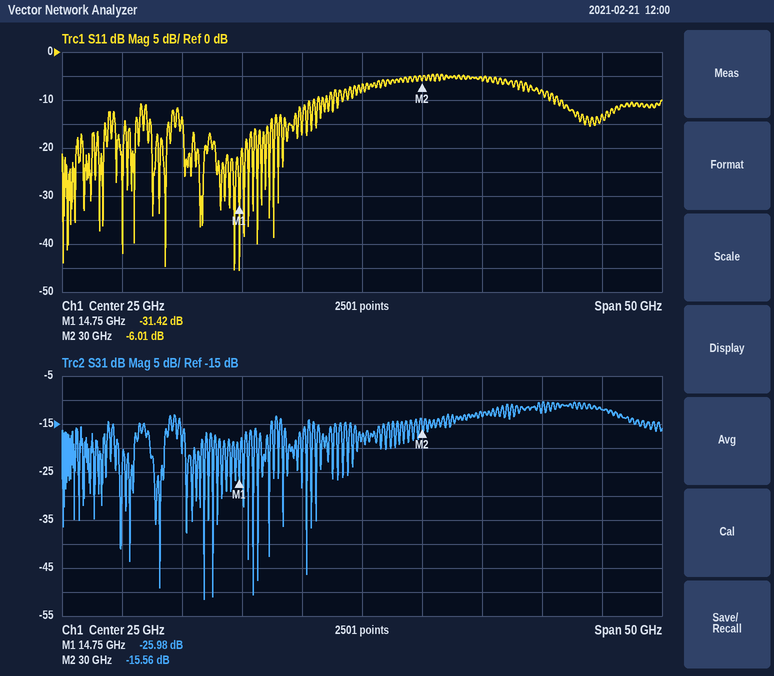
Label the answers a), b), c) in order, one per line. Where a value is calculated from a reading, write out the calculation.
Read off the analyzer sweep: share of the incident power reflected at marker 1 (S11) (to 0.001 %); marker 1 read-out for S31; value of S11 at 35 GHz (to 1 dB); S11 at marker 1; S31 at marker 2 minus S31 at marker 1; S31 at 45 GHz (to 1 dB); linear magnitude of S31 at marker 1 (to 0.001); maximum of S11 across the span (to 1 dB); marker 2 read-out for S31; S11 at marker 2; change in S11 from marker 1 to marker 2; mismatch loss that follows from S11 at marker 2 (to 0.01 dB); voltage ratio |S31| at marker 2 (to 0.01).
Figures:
a) 10^(-31.42/10) ≈ 0.072 %
b) -25.98 dB
c) -6 dB
d) -31.42 dB
e) -15.56 − (-25.98) = 10.42 dB
f) -12 dB
g) 10^(-25.98/20) ≈ 0.050
h) -5 dB
i) -15.56 dB
j) -6.01 dB
k) -6.01 − (-31.42) = 25.41 dB
l) −10 log10(1 − 10^(-6.01/10)) ≈ 1.25 dB
m) 10^(-15.56/20) ≈ 0.17
